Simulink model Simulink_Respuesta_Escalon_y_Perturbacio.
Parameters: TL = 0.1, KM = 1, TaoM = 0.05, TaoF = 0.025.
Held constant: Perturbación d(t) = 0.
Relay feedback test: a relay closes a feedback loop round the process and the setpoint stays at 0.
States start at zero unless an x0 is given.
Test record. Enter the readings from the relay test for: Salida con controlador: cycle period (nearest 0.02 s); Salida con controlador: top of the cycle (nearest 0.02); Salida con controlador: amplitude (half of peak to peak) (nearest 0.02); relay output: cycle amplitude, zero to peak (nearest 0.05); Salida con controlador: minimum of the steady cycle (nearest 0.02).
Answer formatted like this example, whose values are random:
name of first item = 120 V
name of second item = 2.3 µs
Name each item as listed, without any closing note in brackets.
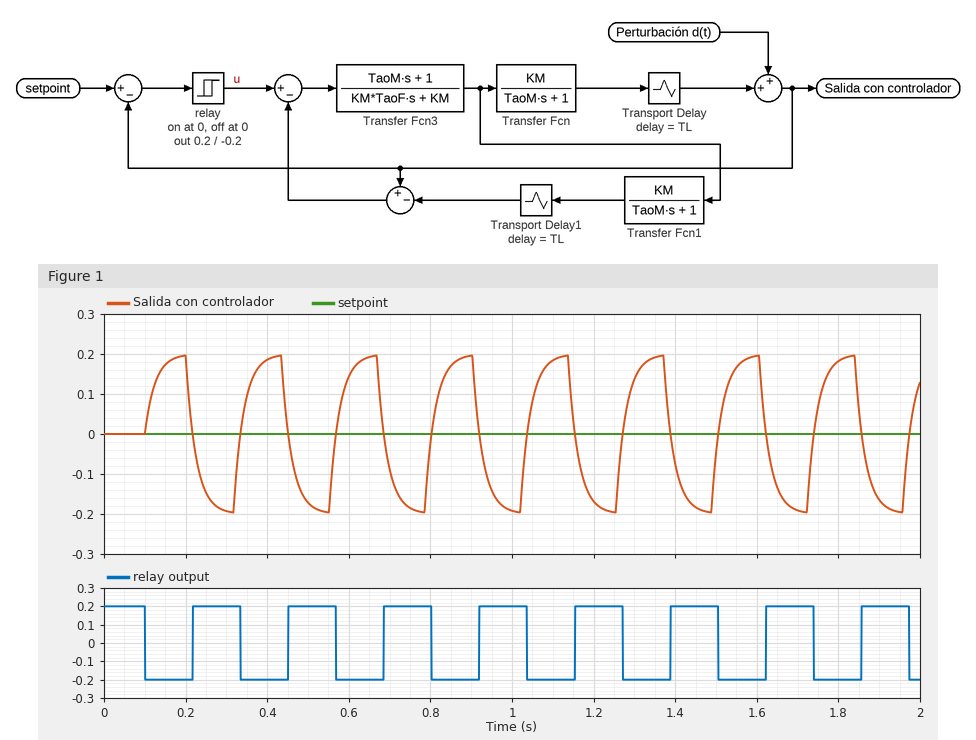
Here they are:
Salida con controlador: cycle period = 0.24 s
Salida con controlador: top of the cycle = 0.20
Salida con controlador: amplitude (half of peak to peak) = 0.20
relay output: cycle amplitude, zero to peak = 0.20
Salida con controlador: minimum of the steady cycle = -0.20
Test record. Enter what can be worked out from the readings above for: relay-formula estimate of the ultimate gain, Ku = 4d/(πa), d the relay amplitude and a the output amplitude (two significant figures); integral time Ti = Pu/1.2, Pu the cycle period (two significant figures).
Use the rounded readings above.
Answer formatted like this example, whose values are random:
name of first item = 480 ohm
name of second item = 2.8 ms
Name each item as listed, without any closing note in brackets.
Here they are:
relay-formula estimate of the ultimate gain, Ku = 4d/(πa), d the relay amplitude and a the output amplitude = 1.3
integral time Ti = Pu/1.2, Pu the cycle period = 0.20 s
